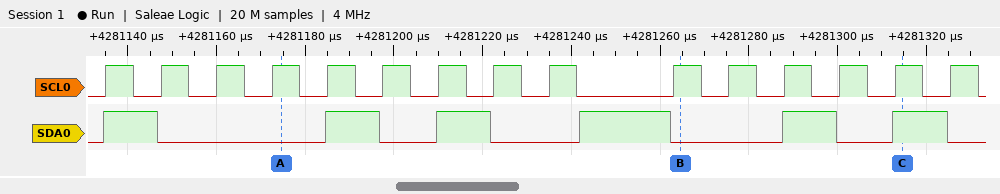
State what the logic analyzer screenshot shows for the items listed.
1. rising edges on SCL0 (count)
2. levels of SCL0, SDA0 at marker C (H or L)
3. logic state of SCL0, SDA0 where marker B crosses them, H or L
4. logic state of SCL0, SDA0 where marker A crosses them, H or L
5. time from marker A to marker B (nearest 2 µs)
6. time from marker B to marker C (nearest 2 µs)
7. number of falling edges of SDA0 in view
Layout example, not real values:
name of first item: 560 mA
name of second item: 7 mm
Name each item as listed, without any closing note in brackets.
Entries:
rising edges on SCL0: 15
levels of SCL0, SDA0 at marker C: SCL0=H, SDA0=H
logic state of SCL0, SDA0 where marker B crosses them, H or L: SCL0=H, SDA0=L
logic state of SCL0, SDA0 where marker A crosses them, H or L: SCL0=H, SDA0=L
time from marker A to marker B: 90 µs
time from marker B to marker C: 50 µs
number of falling edges of SDA0 in view: 6
